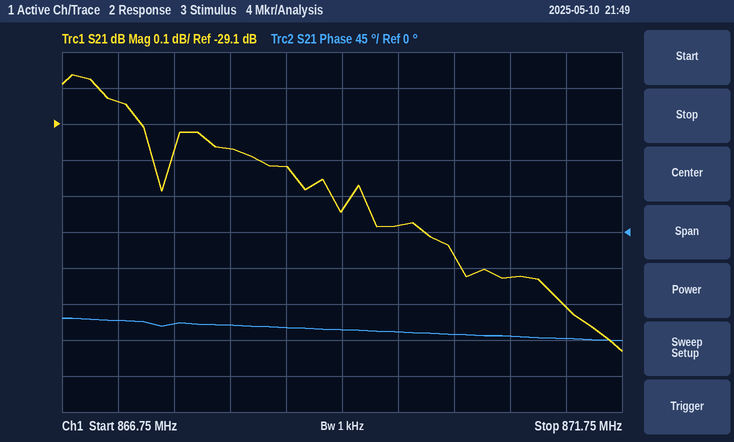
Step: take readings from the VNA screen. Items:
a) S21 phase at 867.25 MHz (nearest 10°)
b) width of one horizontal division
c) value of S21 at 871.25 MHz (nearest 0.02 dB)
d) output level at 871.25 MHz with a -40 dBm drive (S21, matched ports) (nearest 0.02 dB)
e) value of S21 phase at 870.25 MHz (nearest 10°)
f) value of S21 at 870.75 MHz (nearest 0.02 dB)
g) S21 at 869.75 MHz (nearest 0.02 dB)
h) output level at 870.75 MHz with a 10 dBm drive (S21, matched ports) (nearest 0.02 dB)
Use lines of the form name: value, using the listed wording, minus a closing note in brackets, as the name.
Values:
S21 phase at 867.25 MHz: -110°
width of one horizontal division: 500 kHz
value of S21 at 871.25 MHz: -29.60 dB
output level at 871.25 MHz with a -40 dBm drive (S21, matched ports): -69.60 dBm
value of S21 phase at 870.25 MHz: -130°
value of S21 at 870.75 MHz: -29.52 dB
S21 at 869.75 MHz: -29.38 dB
output level at 870.75 MHz with a 10 dBm drive (S21, matched ports): -19.52 dBm
